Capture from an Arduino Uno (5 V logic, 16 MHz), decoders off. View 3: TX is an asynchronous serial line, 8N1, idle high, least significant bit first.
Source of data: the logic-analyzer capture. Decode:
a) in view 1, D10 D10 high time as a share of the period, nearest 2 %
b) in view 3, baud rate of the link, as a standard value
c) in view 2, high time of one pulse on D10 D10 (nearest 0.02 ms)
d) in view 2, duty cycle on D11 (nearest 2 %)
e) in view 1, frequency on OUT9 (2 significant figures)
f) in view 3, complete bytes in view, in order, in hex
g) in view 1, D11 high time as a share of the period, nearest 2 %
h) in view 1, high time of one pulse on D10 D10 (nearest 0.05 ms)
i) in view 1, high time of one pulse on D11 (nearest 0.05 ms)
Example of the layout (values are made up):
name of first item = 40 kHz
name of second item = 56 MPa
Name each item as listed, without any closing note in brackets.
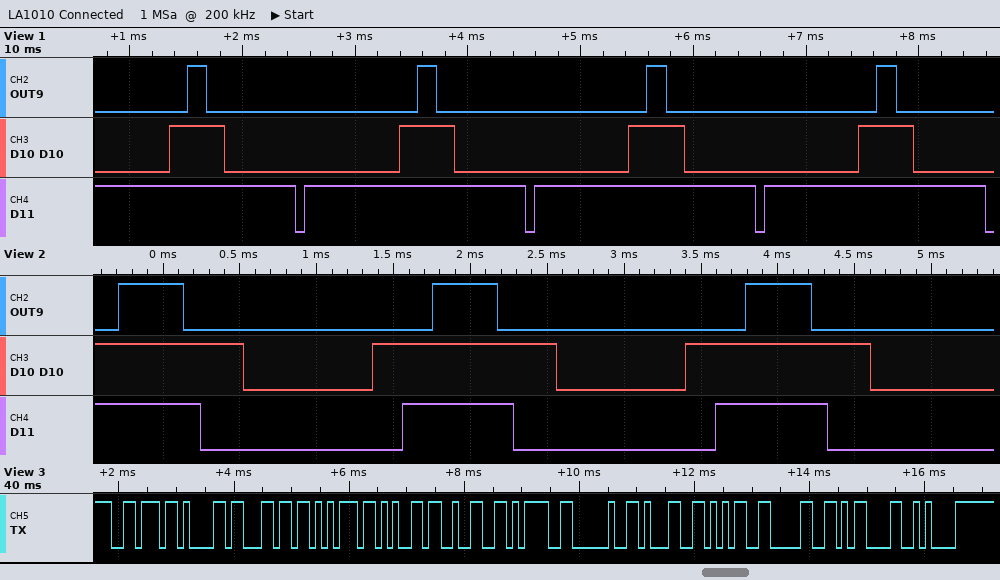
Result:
in view 1, D10 D10 high time as a share of the period, nearest 2 % = 24 %
in view 3, baud rate of the link, as a standard value = 9600 baud
in view 2, high time of one pulse on D10 D10 = 1.20 ms
in view 2, duty cycle on D11 = 36 %
in view 1, frequency on OUT9 = 490 Hz
in view 3, complete bytes in view, in order, in hex = 76 61 6C 75 65 32 3D 20 31 35 30 0D 0A
in view 1, D11 high time as a share of the period, nearest 2 % = 96 %
in view 1, high time of one pulse on D10 D10 = 0.50 ms
in view 1, high time of one pulse on D11 = 1.95 ms
